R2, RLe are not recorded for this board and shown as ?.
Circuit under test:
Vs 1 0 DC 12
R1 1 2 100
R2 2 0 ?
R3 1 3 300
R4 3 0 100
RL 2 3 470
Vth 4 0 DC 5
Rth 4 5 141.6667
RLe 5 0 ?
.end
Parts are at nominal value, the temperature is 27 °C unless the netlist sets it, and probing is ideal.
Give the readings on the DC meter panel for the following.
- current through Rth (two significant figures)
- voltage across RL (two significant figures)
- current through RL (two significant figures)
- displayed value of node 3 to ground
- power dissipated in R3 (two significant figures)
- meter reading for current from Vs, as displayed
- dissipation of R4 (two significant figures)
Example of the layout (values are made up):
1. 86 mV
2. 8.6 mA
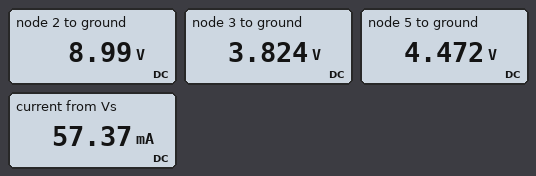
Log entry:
1. 3.7 mA
2. 5.2 V
3. 11 mA
4. 3.824 V
5. 220 mW
6. 57.37 mA
7. 150 mW
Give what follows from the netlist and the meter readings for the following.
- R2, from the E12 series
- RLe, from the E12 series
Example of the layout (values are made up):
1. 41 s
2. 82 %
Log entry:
1. 470 Ω
2. 1.2 kΩ
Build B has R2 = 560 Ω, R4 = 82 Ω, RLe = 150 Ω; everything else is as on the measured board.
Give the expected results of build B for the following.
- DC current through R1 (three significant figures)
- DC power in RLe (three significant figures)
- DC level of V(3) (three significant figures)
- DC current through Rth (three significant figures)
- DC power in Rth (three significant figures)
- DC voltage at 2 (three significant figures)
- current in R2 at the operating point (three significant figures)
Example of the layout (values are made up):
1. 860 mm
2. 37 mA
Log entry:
1. 28.6 mA
2. 44.1 mW
3. 3.37 V
4. 17.1 mA
5. 41.6 mW
6. 9.14 V
7. 16.3 mA
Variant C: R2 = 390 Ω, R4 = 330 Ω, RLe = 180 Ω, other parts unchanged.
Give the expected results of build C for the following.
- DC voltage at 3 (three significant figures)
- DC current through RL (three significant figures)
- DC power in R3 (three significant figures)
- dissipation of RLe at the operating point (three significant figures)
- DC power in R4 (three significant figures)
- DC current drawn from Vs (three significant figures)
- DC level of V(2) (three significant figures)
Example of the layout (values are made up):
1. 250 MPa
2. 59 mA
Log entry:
1. 7.01 V
2. 4.62 mA
3. 82.9 mW
4. 43.5 mW
5. 149 mW
6. 44.8 mA
7. 9.18 V
